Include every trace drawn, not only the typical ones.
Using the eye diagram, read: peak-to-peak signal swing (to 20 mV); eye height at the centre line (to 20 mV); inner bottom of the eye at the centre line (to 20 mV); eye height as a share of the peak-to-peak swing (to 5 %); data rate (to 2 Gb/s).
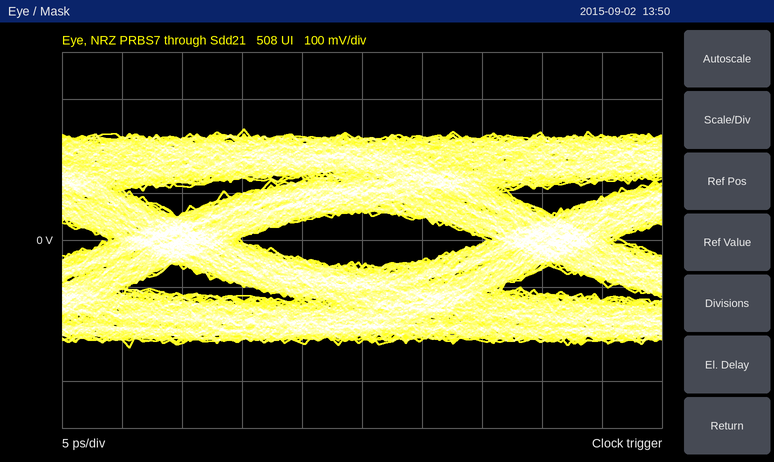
460 mV
120 mV
-60 mV
25 %
32 Gb/s
